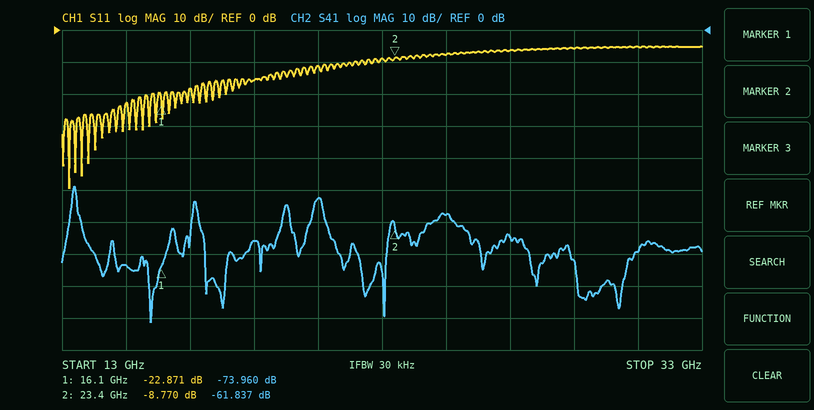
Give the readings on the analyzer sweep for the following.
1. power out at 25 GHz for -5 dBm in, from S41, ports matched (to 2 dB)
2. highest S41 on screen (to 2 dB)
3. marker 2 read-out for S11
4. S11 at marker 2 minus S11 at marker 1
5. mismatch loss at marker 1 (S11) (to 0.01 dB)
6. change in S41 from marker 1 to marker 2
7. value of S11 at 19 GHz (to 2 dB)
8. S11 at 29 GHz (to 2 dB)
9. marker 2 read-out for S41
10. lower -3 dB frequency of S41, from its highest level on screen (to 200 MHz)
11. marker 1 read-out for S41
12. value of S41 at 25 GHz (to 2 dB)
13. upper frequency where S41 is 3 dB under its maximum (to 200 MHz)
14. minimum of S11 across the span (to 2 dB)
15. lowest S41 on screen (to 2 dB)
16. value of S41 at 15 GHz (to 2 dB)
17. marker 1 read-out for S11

-62 dBm
-48 dB
-8.770 dB
14.101 dB
0.02 dB
12.123 dB
-16 dB
-6 dB
-61.837 dB
13.4 GHz
-73.960 dB
-58 dB
13.4 GHz
-50 dB
-92 dB
-74 dB
-22.871 dB
